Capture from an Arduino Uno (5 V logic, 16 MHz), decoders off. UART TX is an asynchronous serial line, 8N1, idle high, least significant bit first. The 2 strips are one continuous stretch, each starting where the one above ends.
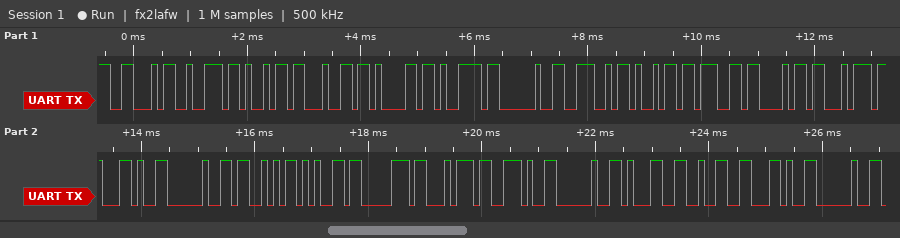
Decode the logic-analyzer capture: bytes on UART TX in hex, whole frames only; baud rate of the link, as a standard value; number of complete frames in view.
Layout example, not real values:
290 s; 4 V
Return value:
46 72 69 64 61 79 20 4E 69 67 68 74 2C 20 53 65 70 74 2E 20 31 32 2C 20; 9600 baud; 24
